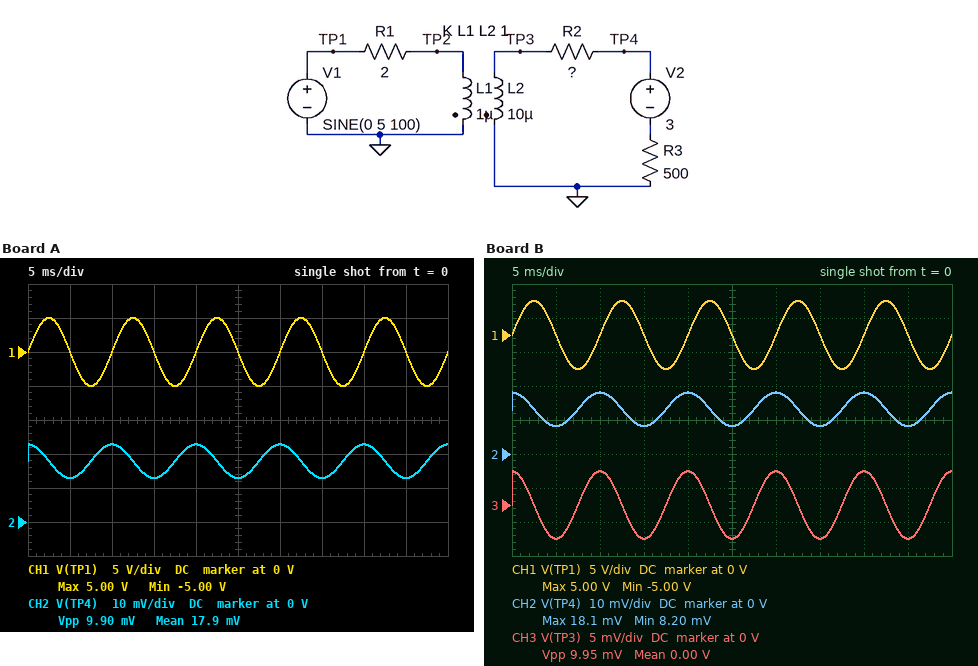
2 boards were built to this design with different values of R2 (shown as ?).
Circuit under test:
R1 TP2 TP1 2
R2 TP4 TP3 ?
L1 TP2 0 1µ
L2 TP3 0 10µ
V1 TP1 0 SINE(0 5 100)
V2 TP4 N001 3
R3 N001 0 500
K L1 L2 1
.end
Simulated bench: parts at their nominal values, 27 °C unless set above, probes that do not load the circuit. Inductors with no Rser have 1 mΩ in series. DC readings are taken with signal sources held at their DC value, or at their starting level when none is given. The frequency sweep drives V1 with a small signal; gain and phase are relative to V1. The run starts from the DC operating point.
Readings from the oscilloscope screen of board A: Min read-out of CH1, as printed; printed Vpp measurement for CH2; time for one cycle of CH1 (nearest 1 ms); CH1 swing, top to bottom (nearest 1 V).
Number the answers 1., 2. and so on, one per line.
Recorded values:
1. -5.00 V
2. 9.90 mV
3. 10 ms
4. 10 V
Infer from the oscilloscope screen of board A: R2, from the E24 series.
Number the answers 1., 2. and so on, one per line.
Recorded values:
1. 3 Ω
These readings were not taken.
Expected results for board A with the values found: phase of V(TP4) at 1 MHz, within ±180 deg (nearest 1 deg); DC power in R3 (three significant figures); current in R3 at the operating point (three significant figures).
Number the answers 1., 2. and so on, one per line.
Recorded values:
1. 17 deg
2. 17.8 mW
3. 5.96 mA
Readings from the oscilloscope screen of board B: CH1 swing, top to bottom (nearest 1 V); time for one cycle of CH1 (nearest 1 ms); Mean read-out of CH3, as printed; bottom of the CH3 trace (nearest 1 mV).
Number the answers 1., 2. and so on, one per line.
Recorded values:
1. 10 V
2. 10 ms
3. 0.00 V
4. -5 mV
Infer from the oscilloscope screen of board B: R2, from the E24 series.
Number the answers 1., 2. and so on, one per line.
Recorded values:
1. 2.2 Ω
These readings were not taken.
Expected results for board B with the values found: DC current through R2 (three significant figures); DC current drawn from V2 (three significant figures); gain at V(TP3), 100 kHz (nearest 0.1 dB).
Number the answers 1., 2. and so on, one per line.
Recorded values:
1. 5.97 mA
2. 5.97 mA
3. -0.5 dB
